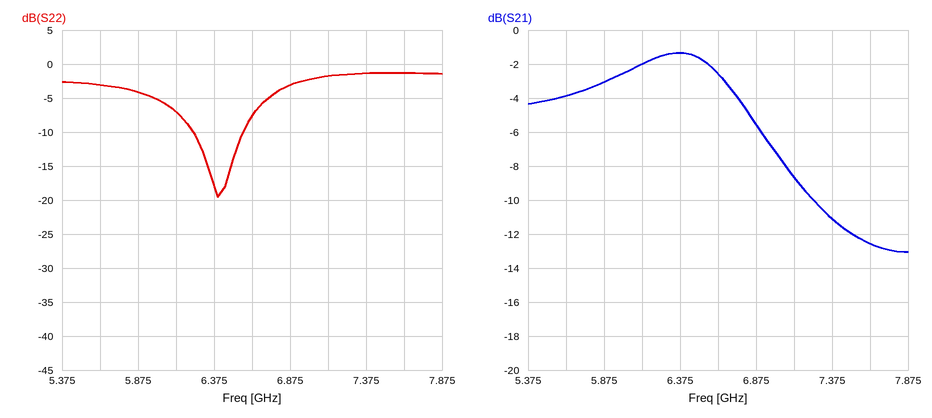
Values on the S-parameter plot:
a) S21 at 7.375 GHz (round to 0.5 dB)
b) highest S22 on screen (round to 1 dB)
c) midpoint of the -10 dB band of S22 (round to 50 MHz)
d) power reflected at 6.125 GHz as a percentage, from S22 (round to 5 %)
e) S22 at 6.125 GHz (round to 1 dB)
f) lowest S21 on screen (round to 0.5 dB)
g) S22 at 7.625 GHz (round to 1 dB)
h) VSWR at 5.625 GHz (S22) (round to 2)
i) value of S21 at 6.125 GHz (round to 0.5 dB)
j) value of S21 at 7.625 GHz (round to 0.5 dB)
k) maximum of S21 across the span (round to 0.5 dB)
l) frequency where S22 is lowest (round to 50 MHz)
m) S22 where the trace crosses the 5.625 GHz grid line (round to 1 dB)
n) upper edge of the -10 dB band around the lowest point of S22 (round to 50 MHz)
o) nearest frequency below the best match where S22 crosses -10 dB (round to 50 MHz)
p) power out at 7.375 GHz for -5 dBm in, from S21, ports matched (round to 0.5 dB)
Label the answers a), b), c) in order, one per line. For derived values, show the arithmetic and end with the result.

a) -11.0 dB
b) -1 dB
c) 6.40 GHz
d) 10^(-7/10) ≈ 20 %
e) -7 dB
f) -13.0 dB
g) -1 dB
h) |Γ| = 10^(-3/20) = 0.7079; VSWR = (1 + 0.7079)/(1 − 0.7079) ≈ 6
i) -2.0 dB
j) -12.5 dB
k) -1.5 dB
l) 6.40 GHz
m) -3 dB
n) 6.55 GHz
o) 6.25 GHz
p) -5 dBm + (-11.0 dB) = -16.0 dBm
